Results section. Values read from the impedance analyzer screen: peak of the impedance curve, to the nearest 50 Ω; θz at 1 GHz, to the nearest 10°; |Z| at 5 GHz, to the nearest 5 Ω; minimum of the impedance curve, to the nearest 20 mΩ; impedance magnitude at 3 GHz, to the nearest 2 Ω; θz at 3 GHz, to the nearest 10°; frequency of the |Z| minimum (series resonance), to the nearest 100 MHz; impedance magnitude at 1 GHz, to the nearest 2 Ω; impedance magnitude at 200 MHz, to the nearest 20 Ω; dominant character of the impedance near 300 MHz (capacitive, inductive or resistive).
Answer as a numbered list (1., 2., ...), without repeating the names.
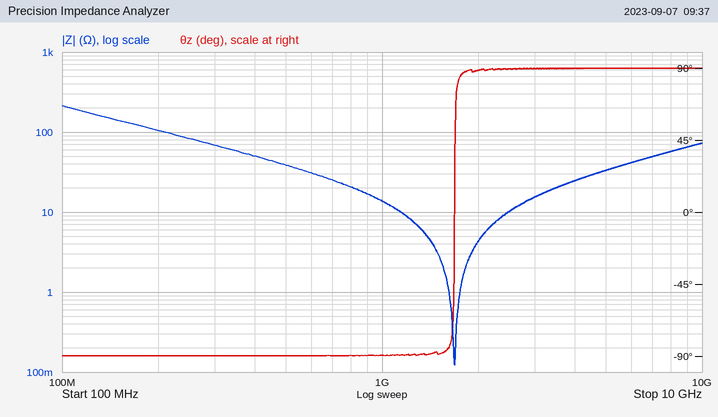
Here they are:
1. 200 Ω
2. -90°
3. 35 Ω
4. 120 mΩ
5. 16 Ω
6. 90°
7. 1.7 GHz
8. 14 Ω
9. 100 Ω
10. capacitive
